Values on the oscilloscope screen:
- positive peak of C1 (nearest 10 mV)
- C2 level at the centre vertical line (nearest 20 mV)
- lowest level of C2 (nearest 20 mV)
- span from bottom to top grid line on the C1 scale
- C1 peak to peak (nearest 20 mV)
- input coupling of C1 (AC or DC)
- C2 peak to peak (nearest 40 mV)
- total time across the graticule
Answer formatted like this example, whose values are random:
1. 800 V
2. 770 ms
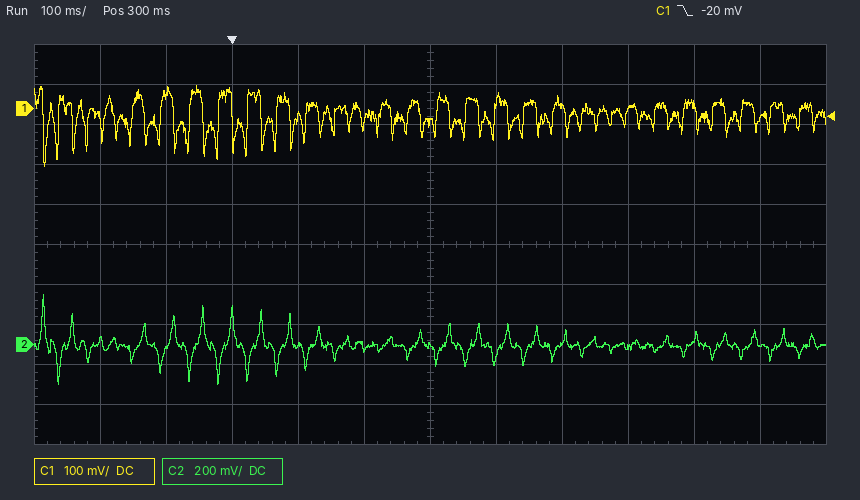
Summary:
1. 60 mV
2. 0 mV
3. -200 mV
4. 1 V
5. 200 mV
6. DC
7. 440 mV
8. 1.2 s
